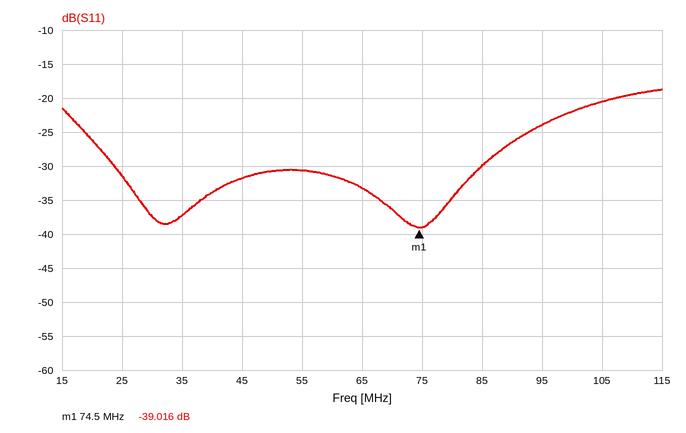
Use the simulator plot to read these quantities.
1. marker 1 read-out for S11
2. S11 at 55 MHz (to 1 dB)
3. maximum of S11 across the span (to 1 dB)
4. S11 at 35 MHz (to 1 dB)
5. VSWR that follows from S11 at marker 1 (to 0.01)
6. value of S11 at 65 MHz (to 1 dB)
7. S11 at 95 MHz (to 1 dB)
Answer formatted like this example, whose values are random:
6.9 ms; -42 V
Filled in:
-39.016 dB; -31 dB; -19 dB; -37 dB; 1.02; -33 dB; -24 dB
